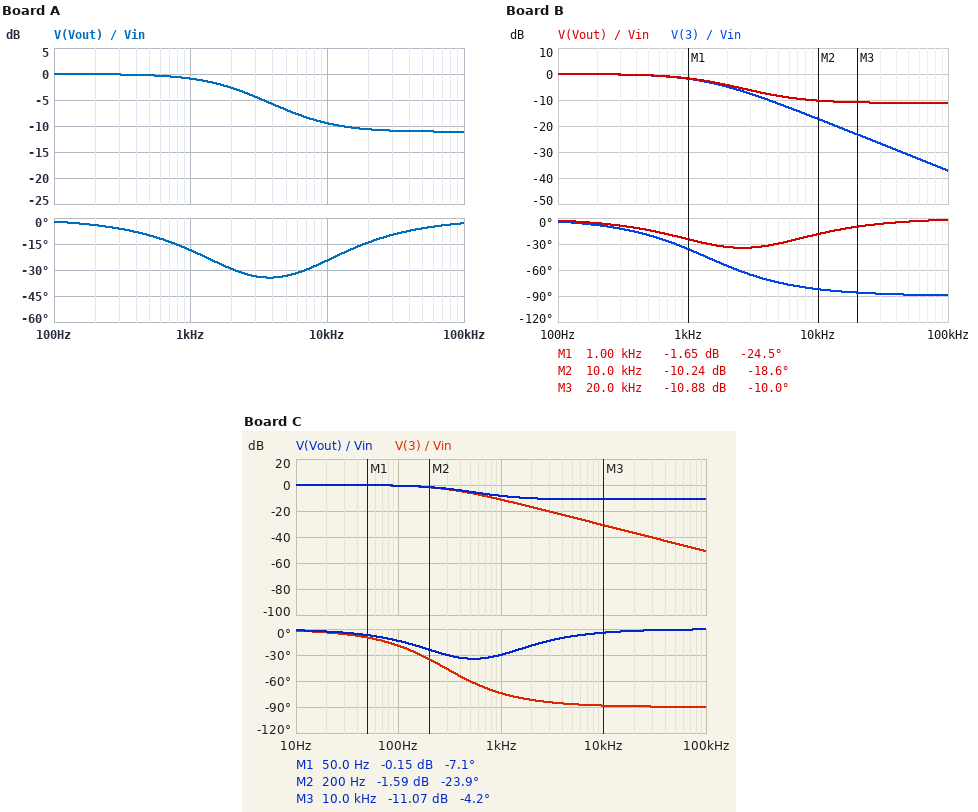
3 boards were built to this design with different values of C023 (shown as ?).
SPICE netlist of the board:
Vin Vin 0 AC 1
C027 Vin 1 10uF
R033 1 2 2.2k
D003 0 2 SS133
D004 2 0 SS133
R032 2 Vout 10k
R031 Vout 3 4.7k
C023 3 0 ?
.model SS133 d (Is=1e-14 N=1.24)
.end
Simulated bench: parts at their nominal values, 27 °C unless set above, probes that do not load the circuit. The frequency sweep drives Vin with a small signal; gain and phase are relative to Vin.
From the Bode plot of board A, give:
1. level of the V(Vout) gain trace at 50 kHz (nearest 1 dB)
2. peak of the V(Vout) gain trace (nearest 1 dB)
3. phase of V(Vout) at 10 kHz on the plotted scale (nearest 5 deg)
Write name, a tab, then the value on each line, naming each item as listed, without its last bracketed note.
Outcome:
level of the V(Vout) gain trace at 50 kHz	-11 dB
peak of the V(Vout) gain trace	0 dB
phase of V(Vout) at 10 kHz on the plotted scale	-25 deg
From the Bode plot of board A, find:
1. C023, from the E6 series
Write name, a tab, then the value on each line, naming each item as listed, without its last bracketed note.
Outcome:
C023, from the E6 series	4.7 nF
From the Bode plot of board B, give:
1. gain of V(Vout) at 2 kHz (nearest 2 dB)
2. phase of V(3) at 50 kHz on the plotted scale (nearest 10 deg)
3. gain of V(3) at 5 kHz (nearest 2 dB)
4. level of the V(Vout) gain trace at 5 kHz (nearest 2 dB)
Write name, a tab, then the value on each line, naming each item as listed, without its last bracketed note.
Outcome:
gain of V(Vout) at 2 kHz	-4 dB
phase of V(3) at 50 kHz on the plotted scale	-90 deg
gain of V(3) at 5 kHz	-12 dB
level of the V(Vout) gain trace at 5 kHz	-8 dB
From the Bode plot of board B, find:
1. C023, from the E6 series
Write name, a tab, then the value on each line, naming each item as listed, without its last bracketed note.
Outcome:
C023, from the E6 series	6.8 nF
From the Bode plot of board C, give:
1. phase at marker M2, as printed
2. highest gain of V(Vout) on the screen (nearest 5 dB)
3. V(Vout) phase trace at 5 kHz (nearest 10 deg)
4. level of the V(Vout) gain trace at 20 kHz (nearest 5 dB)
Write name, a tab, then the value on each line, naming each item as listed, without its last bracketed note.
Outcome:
phase at marker M2, as printed	-23.9 deg
highest gain of V(Vout) on the screen	0 dB
V(Vout) phase trace at 5 kHz	-10 deg
level of the V(Vout) gain trace at 20 kHz	-10 dB
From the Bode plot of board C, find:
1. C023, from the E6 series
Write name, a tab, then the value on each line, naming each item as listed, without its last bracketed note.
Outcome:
C023, from the E6 series	33 nF
